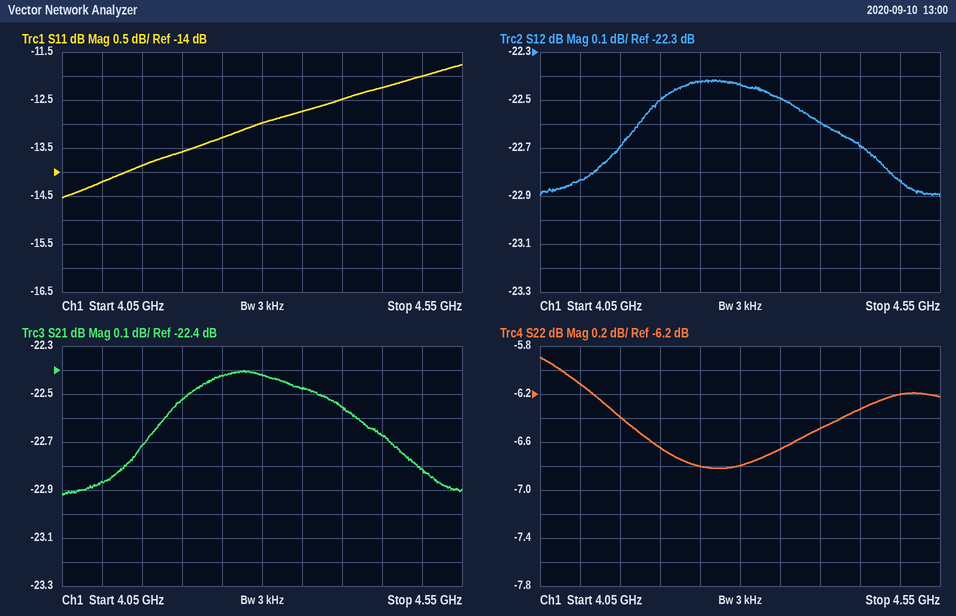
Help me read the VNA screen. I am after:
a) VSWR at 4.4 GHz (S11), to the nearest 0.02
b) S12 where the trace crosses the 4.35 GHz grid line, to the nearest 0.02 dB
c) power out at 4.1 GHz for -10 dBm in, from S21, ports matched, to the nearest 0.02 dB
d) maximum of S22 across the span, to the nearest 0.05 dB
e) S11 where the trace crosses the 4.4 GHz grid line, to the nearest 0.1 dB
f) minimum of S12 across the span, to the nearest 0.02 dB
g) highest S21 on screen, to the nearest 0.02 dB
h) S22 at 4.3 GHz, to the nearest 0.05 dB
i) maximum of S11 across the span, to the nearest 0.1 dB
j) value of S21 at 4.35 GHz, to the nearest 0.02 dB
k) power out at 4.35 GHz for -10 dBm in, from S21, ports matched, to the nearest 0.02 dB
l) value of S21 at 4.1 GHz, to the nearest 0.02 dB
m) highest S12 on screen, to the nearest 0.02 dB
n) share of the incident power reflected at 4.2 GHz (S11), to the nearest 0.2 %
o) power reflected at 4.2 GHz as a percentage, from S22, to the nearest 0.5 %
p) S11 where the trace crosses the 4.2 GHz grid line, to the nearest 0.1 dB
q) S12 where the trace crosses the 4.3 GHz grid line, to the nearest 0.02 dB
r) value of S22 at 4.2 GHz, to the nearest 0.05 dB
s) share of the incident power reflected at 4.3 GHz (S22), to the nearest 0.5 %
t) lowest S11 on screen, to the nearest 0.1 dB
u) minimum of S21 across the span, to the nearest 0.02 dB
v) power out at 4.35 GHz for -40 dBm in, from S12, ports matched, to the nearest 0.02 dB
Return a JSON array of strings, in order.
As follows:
["1.62", "-22.50 dB", "-32.86 dBm", "-5.90 dB", "-12.5 dB", "-22.90 dB", "-22.40 dB", "-6.80 dB", "-11.8 dB", "-22.48 dB", "-32.48 dBm", "-22.86 dB", "-22.42 dB", "4.4 %", "21.5 %", "-13.6 dB", "-22.44 dB", "-6.65 dB", "21.0 %", "-14.5 dB", "-22.92 dB", "-62.50 dBm"]
